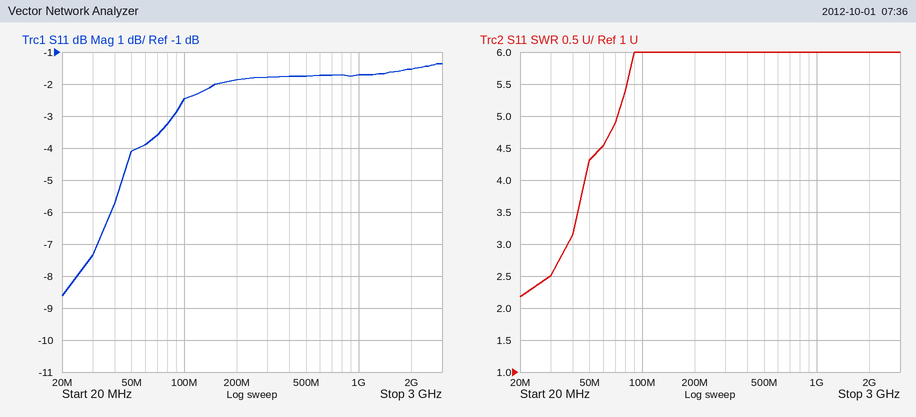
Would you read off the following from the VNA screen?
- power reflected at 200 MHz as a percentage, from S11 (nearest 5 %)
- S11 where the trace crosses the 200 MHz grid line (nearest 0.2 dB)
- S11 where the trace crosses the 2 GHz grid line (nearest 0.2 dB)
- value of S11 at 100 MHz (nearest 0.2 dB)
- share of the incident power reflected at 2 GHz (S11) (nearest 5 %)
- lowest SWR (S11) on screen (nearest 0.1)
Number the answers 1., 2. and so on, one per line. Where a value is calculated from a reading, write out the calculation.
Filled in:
1. 10^(-1.8/10) ≈ 66.1 %, so 65 % to the nearest 5 %
2. -1.8 dB
3. -1.6 dB
4. -2.4 dB
5. 10^(-1.6/10) ≈ 69.2 %, so 70 % to the nearest 5 %
6. 2.2
